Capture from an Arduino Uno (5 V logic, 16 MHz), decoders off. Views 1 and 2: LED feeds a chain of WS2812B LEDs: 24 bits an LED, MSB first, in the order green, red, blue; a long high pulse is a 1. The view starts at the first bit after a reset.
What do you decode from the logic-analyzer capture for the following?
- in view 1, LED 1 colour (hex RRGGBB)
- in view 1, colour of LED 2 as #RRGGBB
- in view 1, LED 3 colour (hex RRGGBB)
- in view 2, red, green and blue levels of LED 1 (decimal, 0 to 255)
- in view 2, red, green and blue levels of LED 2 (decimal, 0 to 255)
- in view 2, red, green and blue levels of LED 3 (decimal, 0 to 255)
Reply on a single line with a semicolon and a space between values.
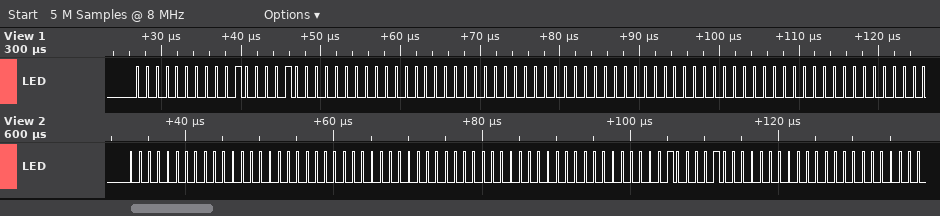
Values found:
#210000; #000000; #000000; 0, 0, 0; 0, 0, 0; 33, 0, 0
